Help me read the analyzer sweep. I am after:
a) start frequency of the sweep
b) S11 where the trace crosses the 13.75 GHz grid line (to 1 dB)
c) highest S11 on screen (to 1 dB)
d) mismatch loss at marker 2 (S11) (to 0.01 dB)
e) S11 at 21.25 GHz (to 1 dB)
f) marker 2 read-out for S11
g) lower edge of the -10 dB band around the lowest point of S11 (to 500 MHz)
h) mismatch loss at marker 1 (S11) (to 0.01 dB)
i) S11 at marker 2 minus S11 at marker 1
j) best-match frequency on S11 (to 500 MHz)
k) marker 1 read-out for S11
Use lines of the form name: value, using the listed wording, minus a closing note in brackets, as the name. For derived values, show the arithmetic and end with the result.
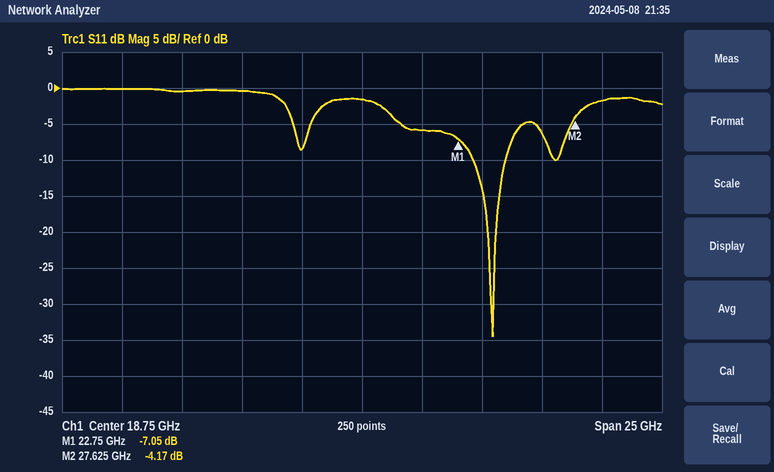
start frequency of the sweep: 6.25 GHz
S11 where the trace crosses the 13.75 GHz grid line: 0 dB
highest S11 on screen: 0 dB
mismatch loss at marker 2 (S11): −10 log10(1 − 10^(-4.17/10)) ≈ 2.10 dB
S11 at 21.25 GHz: -6 dB
marker 2 read-out for S11: -4.17 dB
lower edge of the -10 dB band around the lowest point of S11: 23.5 GHz
mismatch loss at marker 1 (S11): −10 log10(1 − 10^(-7.05/10)) ≈ 0.95 dB
S11 at marker 2 minus S11 at marker 1: -4.17 − (-7.05) = 2.88 dB
best-match frequency on S11: 24.0 GHz
marker 1 read-out for S11: -7.05 dB
